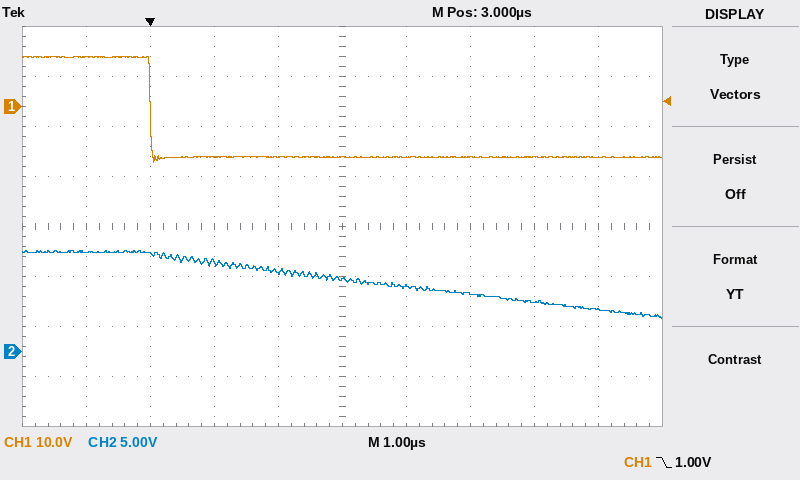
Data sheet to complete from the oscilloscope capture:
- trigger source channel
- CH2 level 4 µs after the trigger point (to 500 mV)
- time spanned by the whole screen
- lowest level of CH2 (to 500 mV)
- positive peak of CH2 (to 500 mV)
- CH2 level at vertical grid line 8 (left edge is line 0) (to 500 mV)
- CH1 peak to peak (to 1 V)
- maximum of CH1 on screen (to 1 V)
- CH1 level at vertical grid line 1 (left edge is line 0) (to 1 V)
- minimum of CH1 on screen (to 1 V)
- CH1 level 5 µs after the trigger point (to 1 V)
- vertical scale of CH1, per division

CH1
6.5 V
10 µs
3.5 V
10.0 V
5.0 V
21 V
10 V
10 V
-11 V
-10 V
10 V
